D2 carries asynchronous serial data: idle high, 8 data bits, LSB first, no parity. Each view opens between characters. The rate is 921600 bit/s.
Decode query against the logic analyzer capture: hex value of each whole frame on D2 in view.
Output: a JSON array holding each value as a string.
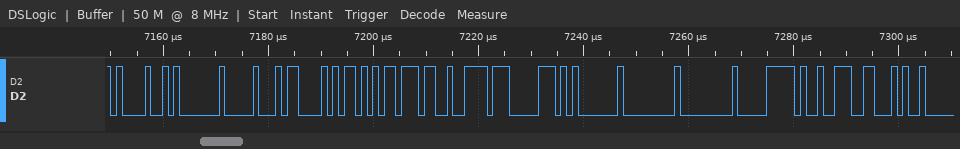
["21, 01, 10, 43, AB, 37, DE, 70, 01, 00, 00, F0, C9, 46"]
